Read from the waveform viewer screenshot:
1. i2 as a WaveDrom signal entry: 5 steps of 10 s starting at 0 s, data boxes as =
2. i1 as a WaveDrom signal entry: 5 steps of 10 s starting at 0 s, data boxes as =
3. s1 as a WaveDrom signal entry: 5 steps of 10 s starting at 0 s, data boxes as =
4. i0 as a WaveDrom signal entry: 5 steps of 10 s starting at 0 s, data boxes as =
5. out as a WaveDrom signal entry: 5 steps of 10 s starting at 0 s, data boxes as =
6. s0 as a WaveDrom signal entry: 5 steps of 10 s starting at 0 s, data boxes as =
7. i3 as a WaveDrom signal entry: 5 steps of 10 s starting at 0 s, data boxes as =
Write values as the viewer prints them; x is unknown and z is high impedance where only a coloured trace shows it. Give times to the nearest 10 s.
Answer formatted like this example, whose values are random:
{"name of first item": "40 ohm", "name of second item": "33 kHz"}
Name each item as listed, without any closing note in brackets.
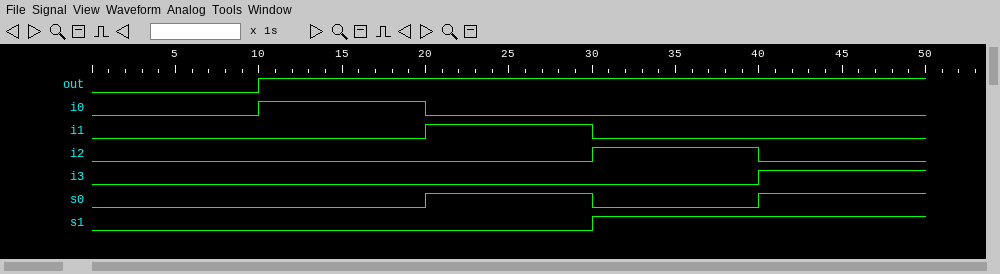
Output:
{"i2 as a WaveDrom signal entry: 5 steps of 10 s starting at 0 s, data boxes as =": "{name: 'i2', wave: '0..10'}", "i1 as a WaveDrom signal entry: 5 steps of 10 s starting at 0 s, data boxes as =": "{name: 'i1', wave: '0.10.'}", "s1 as a WaveDrom signal entry: 5 steps of 10 s starting at 0 s, data boxes as =": "{name: 's1', wave: '0..1.'}", "i0 as a WaveDrom signal entry: 5 steps of 10 s starting at 0 s, data boxes as =": "{name: 'i0', wave: '010..'}", "out as a WaveDrom signal entry: 5 steps of 10 s starting at 0 s, data boxes as =": "{name: 'out', wave: '01...'}", "s0 as a WaveDrom signal entry: 5 steps of 10 s starting at 0 s, data boxes as =": "{name: 's0', wave: '0.101'}", "i3 as a WaveDrom signal entry: 5 steps of 10 s starting at 0 s, data boxes as =": "{name: 'i3', wave: '0...1'}"}
